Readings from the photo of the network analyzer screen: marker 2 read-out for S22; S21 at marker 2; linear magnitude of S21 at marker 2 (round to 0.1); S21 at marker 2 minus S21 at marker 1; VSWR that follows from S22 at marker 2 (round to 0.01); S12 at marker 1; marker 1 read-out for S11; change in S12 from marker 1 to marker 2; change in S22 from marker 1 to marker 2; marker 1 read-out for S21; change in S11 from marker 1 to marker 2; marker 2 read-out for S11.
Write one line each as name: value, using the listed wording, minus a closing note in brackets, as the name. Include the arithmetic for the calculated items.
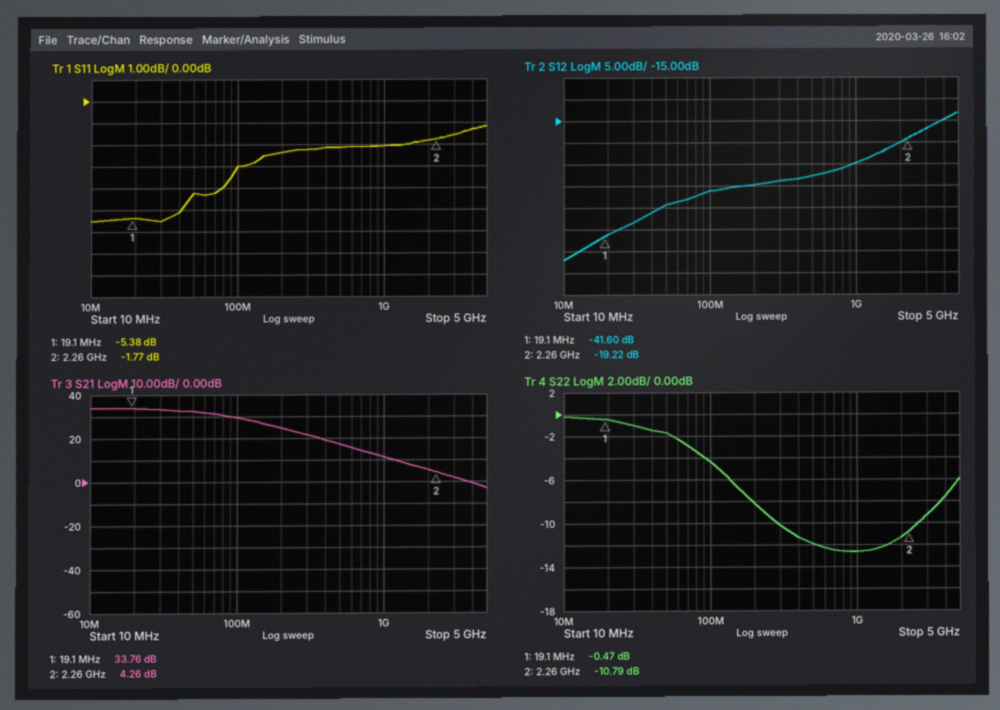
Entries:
marker 2 read-out for S22: -10.79 dB
S21 at marker 2: 4.26 dB
linear magnitude of S21 at marker 2: 10^(4.26/20) ≈ 1.6
S21 at marker 2 minus S21 at marker 1: 4.26 − (33.76) = -29.50 dB
VSWR that follows from S22 at marker 2: (1 + 0.2887)/(1 − 0.2887) ≈ 1.81
S12 at marker 1: -41.60 dB
marker 1 read-out for S11: -5.38 dB
change in S12 from marker 1 to marker 2: -19.22 − (-41.6) = 22.38 dB
change in S22 from marker 1 to marker 2: -10.79 − (-0.47) = -10.32 dB
marker 1 read-out for S21: 33.76 dB
change in S11 from marker 1 to marker 2: -1.77 − (-5.38) = 3.61 dB
marker 2 read-out for S11: -1.77 dB
